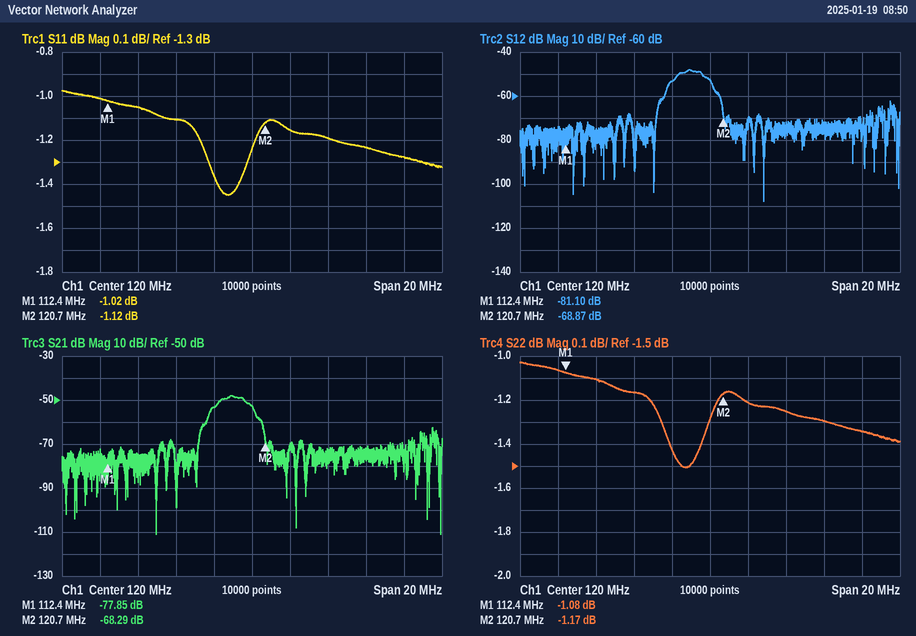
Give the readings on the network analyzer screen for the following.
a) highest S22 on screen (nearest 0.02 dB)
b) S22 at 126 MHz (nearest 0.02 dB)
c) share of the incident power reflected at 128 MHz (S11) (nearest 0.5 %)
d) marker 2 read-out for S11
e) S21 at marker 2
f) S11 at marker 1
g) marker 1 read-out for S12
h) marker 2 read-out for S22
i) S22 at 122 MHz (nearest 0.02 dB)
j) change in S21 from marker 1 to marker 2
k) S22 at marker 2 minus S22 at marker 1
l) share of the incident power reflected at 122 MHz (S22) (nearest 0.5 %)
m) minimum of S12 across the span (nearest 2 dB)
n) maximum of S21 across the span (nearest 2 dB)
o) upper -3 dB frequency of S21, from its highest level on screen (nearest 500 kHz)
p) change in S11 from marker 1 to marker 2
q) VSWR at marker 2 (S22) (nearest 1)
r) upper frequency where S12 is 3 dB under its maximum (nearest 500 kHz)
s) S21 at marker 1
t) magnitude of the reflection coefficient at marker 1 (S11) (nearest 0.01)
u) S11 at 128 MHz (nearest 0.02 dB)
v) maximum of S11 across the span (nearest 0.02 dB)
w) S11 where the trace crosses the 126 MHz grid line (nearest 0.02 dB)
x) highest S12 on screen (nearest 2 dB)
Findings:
-1.02 dB
-1.30 dB
74.5 %
-1.12 dB
-68.29 dB
-1.02 dB
-81.10 dB
-1.17 dB
-1.22 dB
9.56 dB
-0.09 dB
75.5 %
-108 dB
-48 dB
119.5 MHz
-0.10 dB
15
119.5 MHz
-77.85 dB
0.89
-1.28 dB
-0.98 dB
-1.24 dB
-48 dB
